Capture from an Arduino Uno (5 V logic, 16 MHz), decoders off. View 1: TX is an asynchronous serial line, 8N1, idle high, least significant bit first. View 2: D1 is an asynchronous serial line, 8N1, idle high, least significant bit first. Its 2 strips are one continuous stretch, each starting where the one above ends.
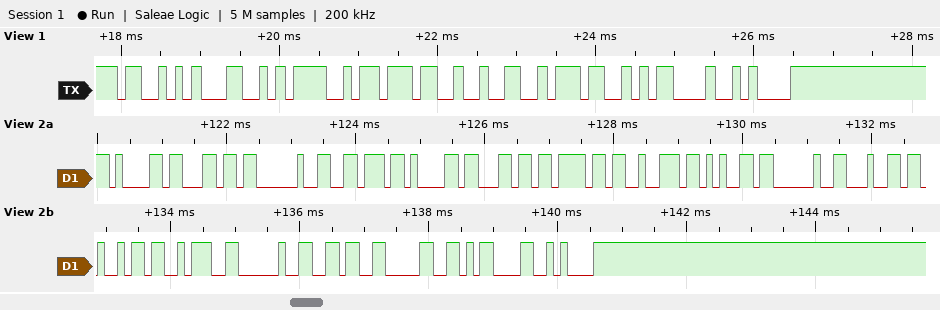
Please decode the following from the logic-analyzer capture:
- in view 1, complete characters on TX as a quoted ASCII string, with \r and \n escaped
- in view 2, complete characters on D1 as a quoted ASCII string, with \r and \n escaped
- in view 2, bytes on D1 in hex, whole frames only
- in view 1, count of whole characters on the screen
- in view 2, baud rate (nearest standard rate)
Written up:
"SLO727\r\n"
"al valore di: 60\r\n"
61 6C 20 76 61 6C 6F 72 65 20 64 69 3A 20 36 30 0D 0A
8
9600 baud
